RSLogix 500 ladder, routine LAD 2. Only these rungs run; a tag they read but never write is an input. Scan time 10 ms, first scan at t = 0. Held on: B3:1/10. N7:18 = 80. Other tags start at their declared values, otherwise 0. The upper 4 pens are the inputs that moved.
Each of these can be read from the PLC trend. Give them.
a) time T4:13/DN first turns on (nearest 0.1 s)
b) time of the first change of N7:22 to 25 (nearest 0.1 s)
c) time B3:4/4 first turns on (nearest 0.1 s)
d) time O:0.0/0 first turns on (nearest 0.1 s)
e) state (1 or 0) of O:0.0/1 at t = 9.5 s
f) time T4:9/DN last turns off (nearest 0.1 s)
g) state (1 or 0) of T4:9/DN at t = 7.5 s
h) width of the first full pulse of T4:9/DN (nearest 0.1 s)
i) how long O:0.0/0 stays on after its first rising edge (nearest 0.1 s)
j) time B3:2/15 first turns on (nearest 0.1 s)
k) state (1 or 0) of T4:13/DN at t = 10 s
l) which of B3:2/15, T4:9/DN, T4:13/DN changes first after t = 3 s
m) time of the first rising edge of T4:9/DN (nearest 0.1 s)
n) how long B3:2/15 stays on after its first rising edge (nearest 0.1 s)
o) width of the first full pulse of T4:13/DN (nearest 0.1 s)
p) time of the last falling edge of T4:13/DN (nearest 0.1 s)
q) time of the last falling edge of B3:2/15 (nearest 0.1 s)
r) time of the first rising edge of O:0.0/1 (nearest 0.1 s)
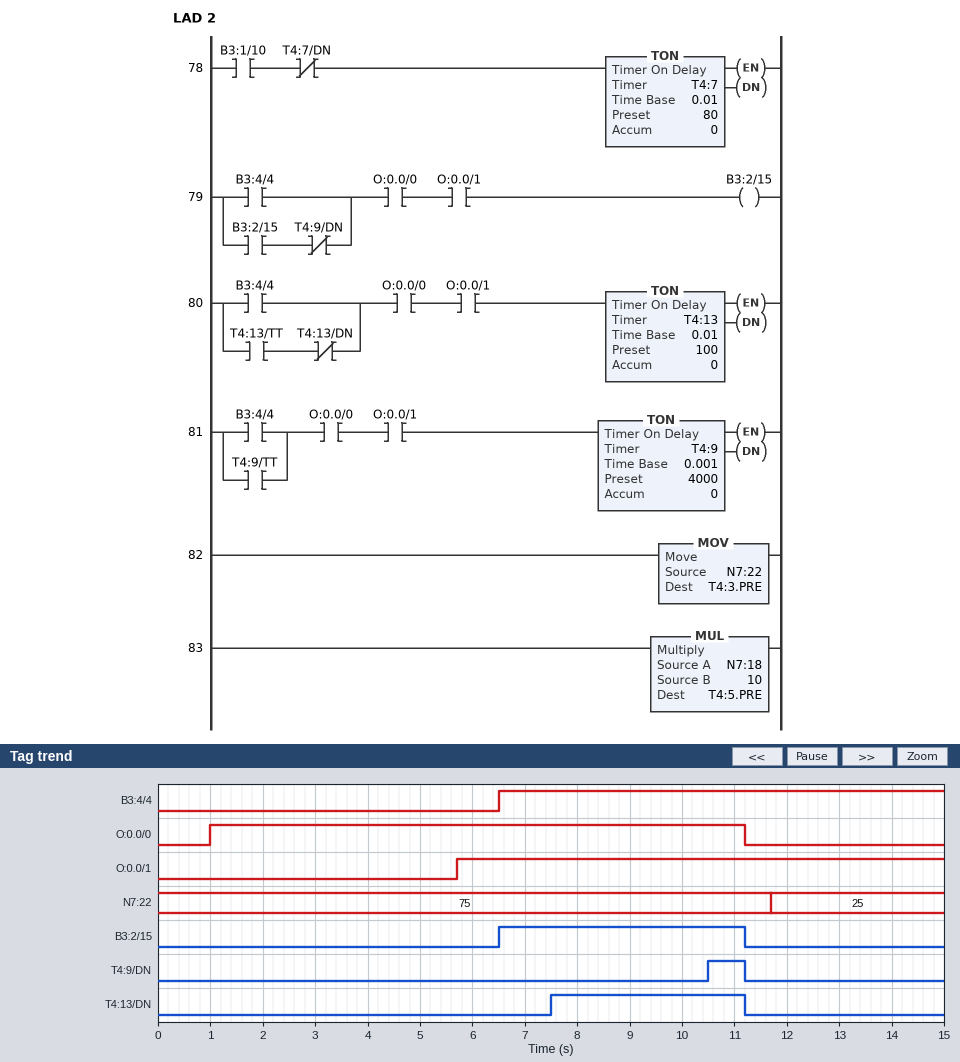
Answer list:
7.5 s
11.7 s
6.5 s
1.0 s
1
11.2 s
0
0.7 s
10.2 s
6.5 s
1
B3:2/15
10.5 s
4.7 s
3.7 s
11.2 s
11.2 s
5.7 s
